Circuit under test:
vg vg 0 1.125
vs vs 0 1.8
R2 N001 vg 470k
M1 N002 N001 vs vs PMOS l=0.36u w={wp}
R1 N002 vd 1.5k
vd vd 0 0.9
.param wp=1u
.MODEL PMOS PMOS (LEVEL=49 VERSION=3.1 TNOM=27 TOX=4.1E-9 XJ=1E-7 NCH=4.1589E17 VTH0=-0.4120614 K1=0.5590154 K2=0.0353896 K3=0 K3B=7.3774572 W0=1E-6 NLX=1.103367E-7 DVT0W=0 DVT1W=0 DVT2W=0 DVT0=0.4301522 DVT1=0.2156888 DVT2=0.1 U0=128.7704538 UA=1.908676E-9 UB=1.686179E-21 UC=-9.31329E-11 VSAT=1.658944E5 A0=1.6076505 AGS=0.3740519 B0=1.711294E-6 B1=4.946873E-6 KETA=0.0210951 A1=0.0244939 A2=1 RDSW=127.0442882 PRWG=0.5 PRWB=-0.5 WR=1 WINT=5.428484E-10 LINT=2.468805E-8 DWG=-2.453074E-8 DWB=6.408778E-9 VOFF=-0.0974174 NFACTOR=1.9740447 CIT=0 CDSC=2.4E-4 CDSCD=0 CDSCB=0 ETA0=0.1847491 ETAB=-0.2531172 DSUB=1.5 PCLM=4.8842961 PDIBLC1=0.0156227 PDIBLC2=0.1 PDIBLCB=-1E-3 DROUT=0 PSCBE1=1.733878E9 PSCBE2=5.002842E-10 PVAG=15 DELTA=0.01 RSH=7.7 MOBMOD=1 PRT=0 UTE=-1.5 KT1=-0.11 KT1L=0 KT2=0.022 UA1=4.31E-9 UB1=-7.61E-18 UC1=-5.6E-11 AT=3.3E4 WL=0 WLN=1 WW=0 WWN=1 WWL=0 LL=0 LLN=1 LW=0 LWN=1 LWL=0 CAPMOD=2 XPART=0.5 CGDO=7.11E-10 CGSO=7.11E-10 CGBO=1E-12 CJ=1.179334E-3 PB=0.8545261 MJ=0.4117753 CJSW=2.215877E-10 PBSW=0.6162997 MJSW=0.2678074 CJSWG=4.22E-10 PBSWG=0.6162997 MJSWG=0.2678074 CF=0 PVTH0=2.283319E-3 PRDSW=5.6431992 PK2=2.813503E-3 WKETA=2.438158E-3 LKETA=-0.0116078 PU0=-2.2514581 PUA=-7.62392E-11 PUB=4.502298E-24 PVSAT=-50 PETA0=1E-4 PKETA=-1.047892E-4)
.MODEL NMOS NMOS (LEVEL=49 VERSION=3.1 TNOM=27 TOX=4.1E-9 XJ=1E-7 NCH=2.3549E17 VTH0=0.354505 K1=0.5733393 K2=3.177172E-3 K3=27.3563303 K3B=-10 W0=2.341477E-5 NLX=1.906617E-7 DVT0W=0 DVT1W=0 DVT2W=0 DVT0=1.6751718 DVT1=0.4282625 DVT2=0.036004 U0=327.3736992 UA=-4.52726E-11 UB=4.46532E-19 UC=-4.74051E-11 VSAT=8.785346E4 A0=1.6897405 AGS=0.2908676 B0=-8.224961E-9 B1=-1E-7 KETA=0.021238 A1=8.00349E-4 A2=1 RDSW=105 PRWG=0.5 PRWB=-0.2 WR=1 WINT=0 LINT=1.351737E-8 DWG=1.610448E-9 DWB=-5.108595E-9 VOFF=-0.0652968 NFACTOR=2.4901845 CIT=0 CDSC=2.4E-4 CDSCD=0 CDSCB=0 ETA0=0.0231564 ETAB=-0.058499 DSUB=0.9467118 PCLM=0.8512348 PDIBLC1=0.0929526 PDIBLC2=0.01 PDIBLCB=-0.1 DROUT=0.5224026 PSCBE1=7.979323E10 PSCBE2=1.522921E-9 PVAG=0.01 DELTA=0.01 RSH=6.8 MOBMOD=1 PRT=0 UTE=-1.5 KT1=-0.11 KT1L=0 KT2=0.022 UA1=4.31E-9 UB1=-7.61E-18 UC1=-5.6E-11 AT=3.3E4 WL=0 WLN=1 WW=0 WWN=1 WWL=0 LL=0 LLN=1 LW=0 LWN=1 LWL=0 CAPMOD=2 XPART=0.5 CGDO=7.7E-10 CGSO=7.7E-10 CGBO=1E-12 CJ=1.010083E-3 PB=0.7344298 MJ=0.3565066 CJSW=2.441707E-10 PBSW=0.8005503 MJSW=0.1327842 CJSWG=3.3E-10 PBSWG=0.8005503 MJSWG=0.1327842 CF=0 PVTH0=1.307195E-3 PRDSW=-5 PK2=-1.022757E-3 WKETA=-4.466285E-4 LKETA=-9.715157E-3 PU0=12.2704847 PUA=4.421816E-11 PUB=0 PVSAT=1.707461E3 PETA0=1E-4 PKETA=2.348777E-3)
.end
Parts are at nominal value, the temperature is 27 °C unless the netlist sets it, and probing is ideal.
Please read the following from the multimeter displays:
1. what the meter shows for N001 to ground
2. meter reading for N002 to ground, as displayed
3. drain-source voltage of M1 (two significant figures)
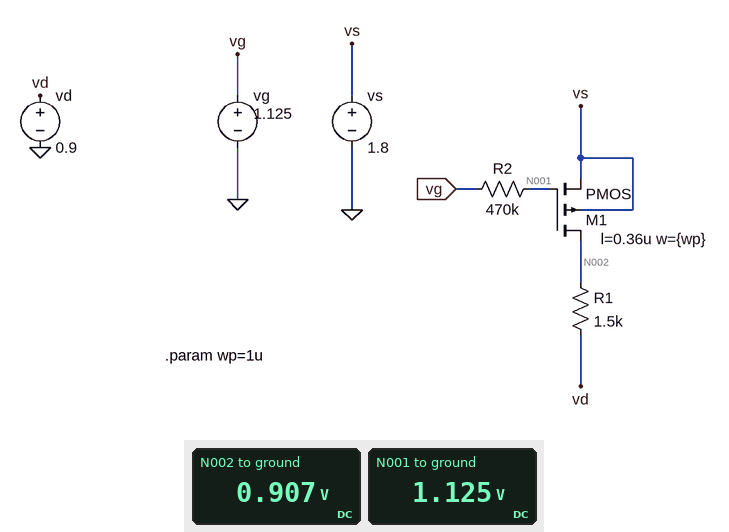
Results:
1.125 V
0.907 V
-890 mV
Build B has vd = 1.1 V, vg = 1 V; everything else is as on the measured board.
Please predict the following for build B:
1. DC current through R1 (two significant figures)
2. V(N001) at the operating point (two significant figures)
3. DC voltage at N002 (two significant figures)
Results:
10 µA
1.0 V
1.1 V
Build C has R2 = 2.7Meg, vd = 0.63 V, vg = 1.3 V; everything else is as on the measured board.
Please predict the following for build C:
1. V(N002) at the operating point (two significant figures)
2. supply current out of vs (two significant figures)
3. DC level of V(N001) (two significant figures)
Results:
630 mV
390 nA
1.3 V
